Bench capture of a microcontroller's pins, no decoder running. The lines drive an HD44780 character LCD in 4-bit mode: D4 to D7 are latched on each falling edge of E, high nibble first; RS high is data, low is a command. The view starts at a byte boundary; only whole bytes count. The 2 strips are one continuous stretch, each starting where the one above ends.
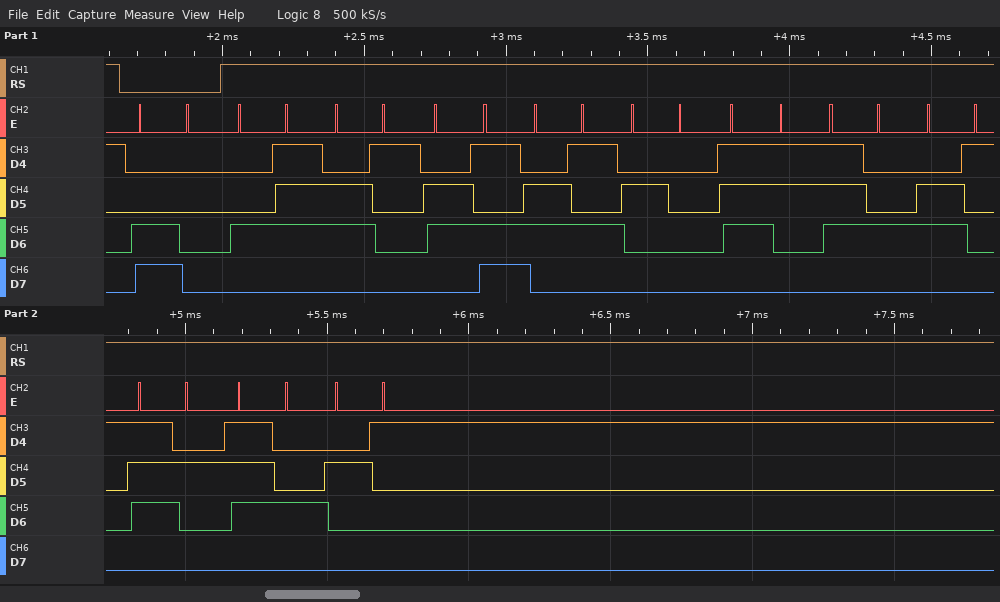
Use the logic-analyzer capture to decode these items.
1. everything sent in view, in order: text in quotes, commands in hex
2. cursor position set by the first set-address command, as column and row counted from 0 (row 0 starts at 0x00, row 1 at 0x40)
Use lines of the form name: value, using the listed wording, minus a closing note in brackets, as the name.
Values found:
everything sent in view, in order: text in quotes, commands in hex: 0xC0 "Game start!"
cursor position set by the first set-address command, as column and row counted from 0: column 0, row 1
